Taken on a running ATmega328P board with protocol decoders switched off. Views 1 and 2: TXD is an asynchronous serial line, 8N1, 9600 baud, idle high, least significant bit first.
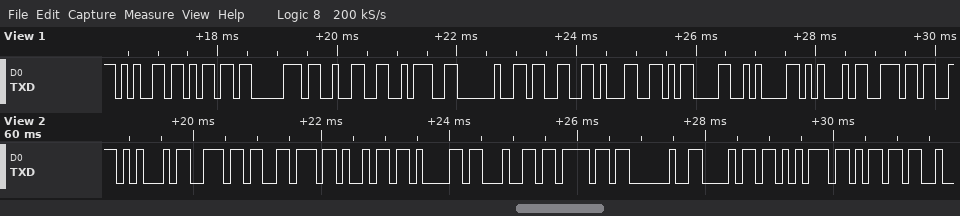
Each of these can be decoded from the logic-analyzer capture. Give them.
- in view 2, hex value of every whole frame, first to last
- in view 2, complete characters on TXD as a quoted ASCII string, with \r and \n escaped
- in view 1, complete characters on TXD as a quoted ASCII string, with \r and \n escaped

0x45 0x6E 0x76 0x69 0x61 0x64 0x6F 0x20 0x68 0x75 0x6D
"Enviado hum"
"emp2: 31\r\nEn"
